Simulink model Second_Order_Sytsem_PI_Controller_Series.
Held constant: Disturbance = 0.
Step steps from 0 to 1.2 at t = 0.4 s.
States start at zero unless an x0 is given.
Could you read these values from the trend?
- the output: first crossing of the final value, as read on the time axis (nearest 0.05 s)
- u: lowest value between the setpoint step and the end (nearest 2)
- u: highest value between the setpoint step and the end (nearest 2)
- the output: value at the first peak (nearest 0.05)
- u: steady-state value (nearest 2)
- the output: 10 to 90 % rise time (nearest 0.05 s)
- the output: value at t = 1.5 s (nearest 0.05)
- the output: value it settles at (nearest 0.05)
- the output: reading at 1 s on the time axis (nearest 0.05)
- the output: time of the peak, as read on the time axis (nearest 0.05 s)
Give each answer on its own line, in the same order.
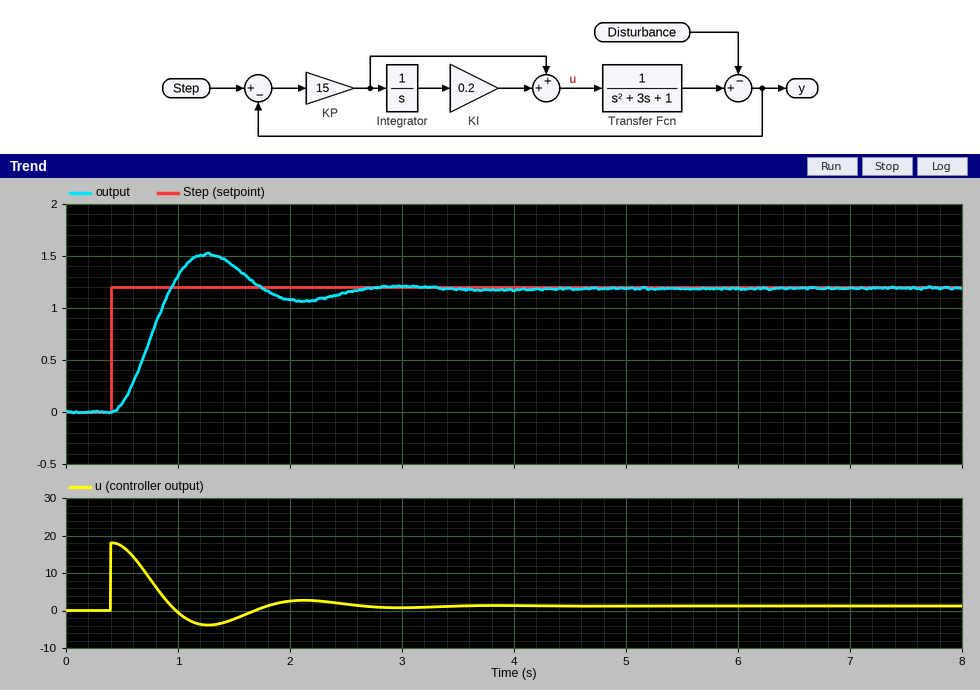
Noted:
0.95 s
-4
18
1.50
2
0.35 s
1.40
1.20
1.30
1.25 s
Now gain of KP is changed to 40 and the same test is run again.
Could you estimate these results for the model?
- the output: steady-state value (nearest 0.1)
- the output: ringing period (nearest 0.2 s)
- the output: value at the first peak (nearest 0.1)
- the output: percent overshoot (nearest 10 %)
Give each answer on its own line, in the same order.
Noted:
1.2
1.0 s
1.8
50 %
